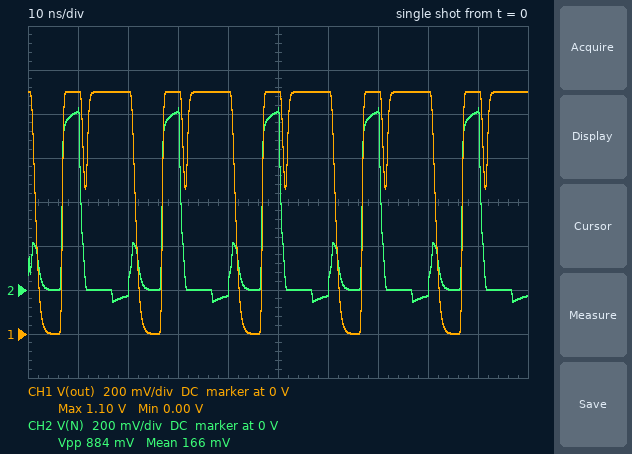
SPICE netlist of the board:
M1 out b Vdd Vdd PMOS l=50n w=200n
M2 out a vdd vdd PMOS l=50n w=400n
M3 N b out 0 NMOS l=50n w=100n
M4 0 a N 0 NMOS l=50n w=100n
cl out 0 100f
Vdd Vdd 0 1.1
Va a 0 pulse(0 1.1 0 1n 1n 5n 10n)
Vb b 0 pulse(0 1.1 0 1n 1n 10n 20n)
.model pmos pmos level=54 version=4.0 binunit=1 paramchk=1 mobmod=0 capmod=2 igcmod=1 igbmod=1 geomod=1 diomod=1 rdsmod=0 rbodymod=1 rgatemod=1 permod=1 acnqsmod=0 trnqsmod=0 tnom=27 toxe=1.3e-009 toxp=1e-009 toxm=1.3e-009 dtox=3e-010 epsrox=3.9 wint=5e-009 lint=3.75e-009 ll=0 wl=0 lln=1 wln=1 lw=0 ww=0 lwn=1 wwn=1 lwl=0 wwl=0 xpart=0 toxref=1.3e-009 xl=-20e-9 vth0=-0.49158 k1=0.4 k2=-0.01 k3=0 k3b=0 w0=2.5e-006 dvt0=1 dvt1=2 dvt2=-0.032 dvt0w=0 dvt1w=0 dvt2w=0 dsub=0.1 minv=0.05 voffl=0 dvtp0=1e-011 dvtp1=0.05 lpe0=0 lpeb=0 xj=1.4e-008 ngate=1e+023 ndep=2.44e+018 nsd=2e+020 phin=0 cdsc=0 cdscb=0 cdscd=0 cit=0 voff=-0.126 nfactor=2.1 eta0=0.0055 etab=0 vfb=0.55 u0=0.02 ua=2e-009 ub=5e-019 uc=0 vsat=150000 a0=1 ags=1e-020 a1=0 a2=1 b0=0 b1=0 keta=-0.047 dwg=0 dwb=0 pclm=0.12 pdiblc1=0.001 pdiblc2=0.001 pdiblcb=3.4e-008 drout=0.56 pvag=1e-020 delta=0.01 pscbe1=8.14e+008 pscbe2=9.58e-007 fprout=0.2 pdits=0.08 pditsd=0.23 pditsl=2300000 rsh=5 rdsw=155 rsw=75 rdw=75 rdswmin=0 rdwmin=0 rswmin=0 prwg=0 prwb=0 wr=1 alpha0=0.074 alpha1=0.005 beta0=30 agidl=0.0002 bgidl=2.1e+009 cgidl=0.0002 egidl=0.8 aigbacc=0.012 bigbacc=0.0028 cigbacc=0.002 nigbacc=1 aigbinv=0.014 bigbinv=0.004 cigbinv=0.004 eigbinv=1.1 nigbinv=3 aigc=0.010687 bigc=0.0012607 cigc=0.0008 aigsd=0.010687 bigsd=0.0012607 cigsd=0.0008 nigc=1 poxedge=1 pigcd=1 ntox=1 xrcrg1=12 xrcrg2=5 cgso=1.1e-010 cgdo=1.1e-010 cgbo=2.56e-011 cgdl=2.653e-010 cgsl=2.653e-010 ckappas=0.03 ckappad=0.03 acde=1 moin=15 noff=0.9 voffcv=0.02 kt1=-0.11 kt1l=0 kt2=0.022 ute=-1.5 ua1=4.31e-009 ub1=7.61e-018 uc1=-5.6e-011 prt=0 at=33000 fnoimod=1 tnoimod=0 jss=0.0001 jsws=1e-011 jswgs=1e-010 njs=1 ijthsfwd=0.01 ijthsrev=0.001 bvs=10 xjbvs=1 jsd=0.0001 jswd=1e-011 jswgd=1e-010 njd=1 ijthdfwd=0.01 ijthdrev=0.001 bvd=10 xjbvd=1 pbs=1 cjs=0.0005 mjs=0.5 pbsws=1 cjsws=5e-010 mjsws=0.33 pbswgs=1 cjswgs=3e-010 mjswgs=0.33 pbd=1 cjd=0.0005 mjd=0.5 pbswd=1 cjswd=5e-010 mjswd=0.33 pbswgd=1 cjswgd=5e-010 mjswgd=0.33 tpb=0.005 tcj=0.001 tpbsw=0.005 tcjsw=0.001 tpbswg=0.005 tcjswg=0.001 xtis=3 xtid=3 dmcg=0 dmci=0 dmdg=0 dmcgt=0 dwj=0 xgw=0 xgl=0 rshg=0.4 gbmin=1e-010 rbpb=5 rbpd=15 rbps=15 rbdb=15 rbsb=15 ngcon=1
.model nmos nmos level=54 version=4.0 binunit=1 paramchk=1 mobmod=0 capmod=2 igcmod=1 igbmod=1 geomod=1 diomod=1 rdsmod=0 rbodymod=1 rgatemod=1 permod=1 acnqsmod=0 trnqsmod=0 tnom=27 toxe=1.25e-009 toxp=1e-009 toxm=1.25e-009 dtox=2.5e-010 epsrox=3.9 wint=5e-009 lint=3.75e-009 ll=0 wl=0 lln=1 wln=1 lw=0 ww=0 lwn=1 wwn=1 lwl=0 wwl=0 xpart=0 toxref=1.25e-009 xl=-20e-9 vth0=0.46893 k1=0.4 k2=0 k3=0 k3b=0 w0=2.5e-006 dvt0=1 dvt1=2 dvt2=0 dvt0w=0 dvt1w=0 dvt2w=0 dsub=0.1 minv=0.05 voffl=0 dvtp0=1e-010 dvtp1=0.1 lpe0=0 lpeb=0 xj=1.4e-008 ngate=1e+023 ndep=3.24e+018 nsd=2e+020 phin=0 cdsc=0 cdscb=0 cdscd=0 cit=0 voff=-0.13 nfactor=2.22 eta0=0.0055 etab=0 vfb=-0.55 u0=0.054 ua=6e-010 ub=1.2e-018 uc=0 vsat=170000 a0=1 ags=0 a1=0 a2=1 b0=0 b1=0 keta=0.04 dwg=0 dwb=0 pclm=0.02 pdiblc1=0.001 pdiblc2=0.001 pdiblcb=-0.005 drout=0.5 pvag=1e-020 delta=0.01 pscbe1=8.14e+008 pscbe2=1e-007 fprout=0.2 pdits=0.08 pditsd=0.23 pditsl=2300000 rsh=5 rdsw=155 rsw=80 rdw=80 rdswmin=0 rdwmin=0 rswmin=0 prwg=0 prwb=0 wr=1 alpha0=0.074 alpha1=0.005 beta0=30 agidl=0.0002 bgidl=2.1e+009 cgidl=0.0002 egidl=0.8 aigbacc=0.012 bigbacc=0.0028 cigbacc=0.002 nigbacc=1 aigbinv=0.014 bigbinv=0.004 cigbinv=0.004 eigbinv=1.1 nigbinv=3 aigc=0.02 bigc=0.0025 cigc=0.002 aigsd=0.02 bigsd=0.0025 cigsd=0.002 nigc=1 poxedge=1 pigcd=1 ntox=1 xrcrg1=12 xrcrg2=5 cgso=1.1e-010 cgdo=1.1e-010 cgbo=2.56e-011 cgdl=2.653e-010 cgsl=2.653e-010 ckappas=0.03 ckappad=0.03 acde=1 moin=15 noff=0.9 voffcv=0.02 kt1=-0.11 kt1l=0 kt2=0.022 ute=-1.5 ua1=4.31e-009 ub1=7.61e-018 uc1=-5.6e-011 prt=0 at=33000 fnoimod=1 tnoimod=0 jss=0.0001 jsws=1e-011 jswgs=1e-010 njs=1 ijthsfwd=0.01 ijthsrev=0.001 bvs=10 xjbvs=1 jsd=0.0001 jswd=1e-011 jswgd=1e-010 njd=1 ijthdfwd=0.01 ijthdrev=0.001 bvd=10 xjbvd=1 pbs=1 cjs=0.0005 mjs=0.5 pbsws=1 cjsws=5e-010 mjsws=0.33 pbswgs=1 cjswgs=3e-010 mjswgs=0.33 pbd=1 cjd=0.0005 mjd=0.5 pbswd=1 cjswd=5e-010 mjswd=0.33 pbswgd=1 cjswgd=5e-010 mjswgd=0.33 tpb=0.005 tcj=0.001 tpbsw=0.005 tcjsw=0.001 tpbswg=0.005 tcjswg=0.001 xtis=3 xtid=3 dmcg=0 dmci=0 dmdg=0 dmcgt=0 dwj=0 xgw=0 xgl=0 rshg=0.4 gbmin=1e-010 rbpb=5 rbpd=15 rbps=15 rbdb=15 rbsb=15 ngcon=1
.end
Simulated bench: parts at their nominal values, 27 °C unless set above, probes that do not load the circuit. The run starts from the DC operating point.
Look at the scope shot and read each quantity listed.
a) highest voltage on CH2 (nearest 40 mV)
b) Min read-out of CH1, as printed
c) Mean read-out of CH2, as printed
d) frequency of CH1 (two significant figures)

840 mV
0.00 V
166 mV
50 MHz
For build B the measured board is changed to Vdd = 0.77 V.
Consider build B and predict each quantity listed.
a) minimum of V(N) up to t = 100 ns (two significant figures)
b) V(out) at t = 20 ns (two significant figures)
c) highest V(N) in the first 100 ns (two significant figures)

-56 mV
770 mV
780 mV
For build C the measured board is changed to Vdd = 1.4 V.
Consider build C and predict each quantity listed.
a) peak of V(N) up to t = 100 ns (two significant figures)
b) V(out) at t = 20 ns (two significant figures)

850 mV
1.4 V
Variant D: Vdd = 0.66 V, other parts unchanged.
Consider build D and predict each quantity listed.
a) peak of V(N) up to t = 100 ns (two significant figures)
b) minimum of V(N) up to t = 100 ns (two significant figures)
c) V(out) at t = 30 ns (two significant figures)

670 mV
-56 mV
660 mV
